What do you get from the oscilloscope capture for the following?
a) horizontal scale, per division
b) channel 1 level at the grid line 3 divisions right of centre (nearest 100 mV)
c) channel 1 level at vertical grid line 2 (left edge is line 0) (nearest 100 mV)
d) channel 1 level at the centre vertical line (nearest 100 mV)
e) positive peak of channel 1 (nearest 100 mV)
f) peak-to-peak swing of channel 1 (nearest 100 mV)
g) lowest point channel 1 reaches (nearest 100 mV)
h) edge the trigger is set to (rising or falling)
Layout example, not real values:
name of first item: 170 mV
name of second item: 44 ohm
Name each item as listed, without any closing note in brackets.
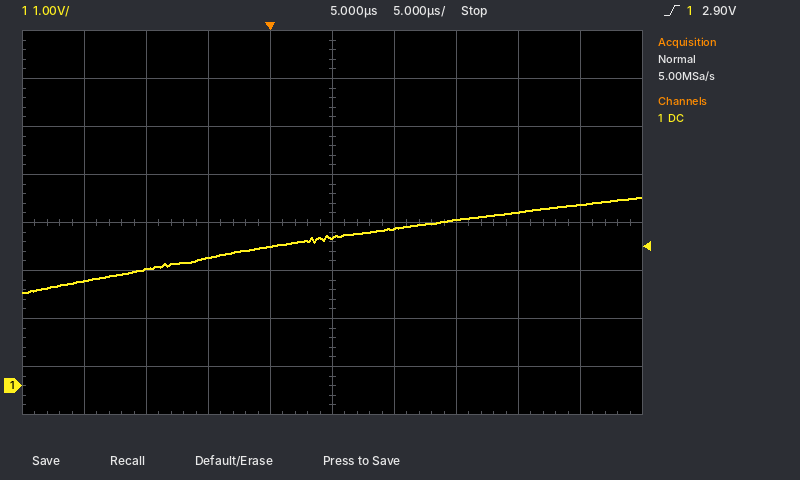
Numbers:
horizontal scale, per division: 5 µs
channel 1 level at the grid line 3 divisions right of centre: 3.6 V
channel 1 level at vertical grid line 2 (left edge is line 0): 2.4 V
channel 1 level at the centre vertical line: 3.1 V
positive peak of channel 1: 3.9 V
peak-to-peak swing of channel 1: 2.0 V
lowest point channel 1 reaches: 1.9 V
edge the trigger is set to: rising
